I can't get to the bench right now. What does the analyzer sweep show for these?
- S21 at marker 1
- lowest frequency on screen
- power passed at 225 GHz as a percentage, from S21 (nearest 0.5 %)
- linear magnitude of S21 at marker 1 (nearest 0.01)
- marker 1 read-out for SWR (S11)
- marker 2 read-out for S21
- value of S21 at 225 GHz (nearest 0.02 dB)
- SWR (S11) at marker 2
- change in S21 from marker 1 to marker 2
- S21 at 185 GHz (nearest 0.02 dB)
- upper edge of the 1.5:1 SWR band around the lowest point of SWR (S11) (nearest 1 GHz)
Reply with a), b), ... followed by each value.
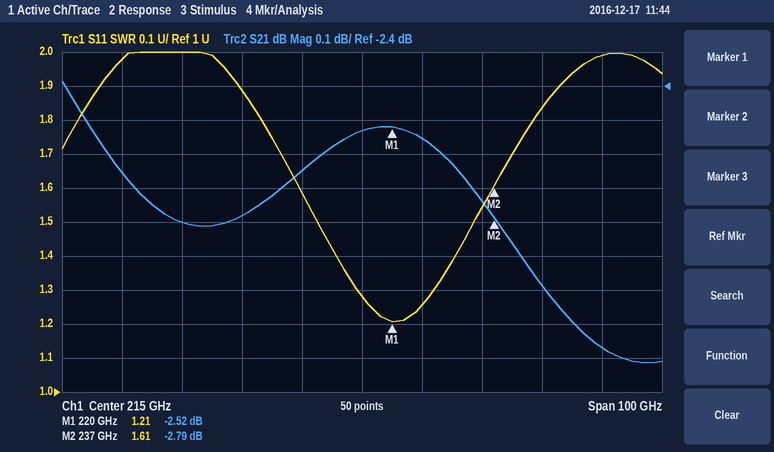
a) -2.52 dB
b) 165 GHz
c) 55.5 %
d) 0.75
e) 1.21
f) -2.79 dB
g) -2.56 dB
h) 1.61
i) -0.27 dB
j) -2.80 dB
k) 234 GHz
